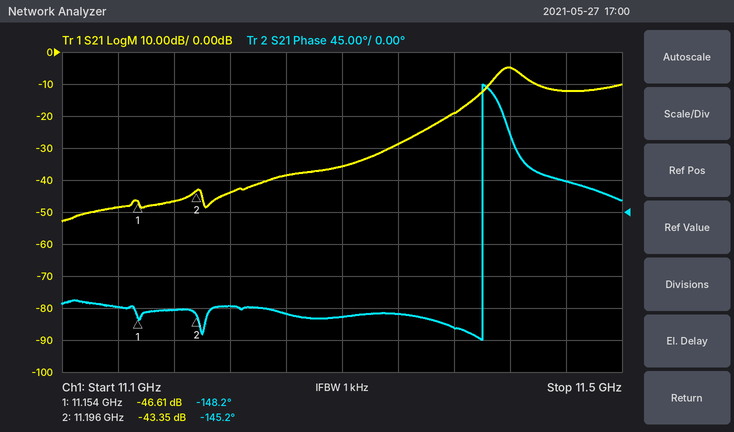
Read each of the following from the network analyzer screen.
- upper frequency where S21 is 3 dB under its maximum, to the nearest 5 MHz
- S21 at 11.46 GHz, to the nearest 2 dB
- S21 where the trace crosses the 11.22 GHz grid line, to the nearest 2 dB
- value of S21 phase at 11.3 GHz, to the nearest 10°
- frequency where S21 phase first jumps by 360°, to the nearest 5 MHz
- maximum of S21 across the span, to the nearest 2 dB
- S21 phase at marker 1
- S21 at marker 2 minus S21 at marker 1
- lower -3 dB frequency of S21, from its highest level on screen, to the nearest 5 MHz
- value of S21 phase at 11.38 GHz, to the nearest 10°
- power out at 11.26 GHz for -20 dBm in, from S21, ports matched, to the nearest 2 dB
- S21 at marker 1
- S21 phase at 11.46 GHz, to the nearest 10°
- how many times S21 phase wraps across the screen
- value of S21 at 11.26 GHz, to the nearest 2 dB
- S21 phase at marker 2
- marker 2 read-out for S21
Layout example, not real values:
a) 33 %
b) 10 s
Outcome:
a) 11.430 GHz
b) -12 dB
c) -44 dB
d) -150°
e) 11.400 GHz
f) -4 dB
g) -148.2°
h) 3.26 dB
i) 11.410 GHz
j) -160°
k) -58 dBm
l) -46.61 dB
m) 40°
n) 1
o) -38 dB
p) -145.2°
q) -43.35 dB
